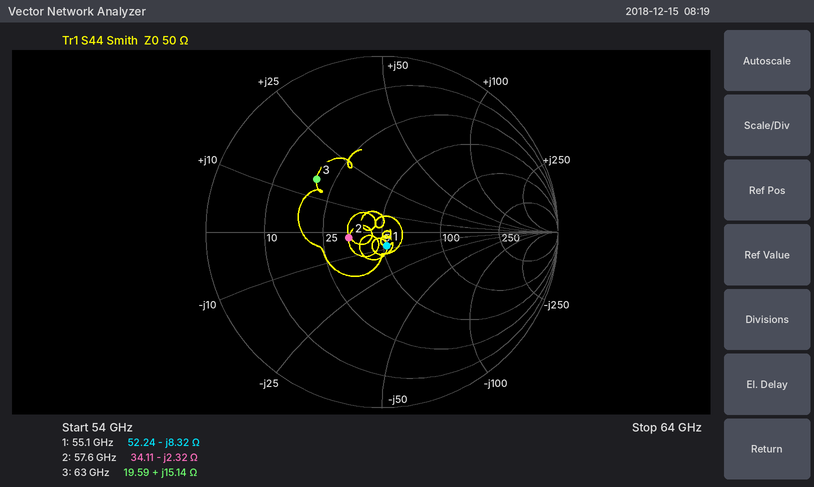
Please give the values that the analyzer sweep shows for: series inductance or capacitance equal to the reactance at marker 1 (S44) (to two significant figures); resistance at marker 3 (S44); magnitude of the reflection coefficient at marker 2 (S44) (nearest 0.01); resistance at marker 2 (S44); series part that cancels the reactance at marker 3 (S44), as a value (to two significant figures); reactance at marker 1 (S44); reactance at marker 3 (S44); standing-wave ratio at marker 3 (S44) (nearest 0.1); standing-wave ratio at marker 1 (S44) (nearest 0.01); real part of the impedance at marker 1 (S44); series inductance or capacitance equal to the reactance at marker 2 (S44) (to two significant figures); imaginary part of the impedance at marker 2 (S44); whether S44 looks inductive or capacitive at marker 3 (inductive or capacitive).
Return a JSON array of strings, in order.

["350 fF", "19.59 Ω", "0.19", "34.11 Ω", "170 fF", "-8.32 Ω", "+15.14 Ω", "2.8", "1.18", "52.24 Ω", "1.2 pF", "-2.32 Ω", "inductive"]
